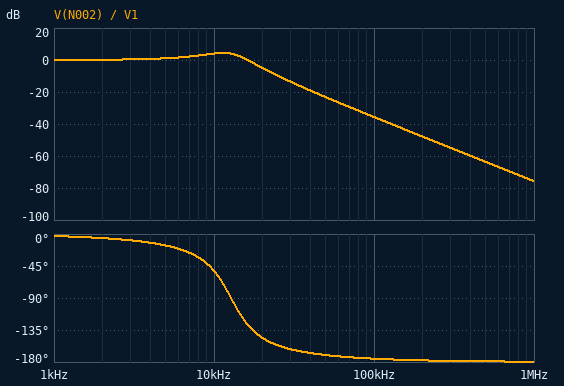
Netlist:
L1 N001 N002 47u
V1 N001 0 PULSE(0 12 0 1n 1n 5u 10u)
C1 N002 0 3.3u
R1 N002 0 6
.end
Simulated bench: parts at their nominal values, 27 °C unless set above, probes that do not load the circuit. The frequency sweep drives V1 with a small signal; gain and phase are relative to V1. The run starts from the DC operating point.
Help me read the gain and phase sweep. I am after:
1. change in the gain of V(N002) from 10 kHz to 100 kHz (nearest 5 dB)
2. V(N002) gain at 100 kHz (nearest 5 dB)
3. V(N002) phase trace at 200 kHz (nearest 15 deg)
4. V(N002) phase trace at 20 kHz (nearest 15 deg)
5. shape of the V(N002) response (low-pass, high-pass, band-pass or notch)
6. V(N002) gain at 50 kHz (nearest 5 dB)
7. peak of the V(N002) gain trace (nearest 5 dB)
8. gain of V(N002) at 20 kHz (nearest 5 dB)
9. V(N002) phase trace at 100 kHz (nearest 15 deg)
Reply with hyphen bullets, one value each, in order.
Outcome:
- -40 dB
- -35 dB
- -180 deg
- -150 deg
- low-pass
- -25 dB
- 5 dB
- -5 dB
- -180 deg
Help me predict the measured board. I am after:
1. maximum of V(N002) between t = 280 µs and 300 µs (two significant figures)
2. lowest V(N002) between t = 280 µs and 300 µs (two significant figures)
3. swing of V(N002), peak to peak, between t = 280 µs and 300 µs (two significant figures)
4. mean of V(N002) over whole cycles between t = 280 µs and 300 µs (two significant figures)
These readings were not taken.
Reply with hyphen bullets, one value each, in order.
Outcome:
- 6.1 V
- 5.9 V
- 250 mV
- 6.0 V
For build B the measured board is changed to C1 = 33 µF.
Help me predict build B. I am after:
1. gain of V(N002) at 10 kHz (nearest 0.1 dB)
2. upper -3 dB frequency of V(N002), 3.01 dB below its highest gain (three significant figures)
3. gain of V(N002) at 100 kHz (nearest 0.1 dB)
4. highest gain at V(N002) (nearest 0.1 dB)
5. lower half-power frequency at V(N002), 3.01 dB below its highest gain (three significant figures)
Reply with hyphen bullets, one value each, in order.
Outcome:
- -14.2 dB
- 4.39 kHz
- -55.7 dB
- 14.1 dB
- 3.57 kHz
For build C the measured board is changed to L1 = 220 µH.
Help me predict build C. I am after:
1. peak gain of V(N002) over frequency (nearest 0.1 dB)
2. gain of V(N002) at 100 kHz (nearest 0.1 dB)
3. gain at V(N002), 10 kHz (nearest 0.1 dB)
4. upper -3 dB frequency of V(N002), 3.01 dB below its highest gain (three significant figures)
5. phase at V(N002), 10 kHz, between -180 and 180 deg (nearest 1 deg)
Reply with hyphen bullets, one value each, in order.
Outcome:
- 0 dB
- -49.1 dB
- -9.4 dB
- 6.11 kHz
- -129 deg
